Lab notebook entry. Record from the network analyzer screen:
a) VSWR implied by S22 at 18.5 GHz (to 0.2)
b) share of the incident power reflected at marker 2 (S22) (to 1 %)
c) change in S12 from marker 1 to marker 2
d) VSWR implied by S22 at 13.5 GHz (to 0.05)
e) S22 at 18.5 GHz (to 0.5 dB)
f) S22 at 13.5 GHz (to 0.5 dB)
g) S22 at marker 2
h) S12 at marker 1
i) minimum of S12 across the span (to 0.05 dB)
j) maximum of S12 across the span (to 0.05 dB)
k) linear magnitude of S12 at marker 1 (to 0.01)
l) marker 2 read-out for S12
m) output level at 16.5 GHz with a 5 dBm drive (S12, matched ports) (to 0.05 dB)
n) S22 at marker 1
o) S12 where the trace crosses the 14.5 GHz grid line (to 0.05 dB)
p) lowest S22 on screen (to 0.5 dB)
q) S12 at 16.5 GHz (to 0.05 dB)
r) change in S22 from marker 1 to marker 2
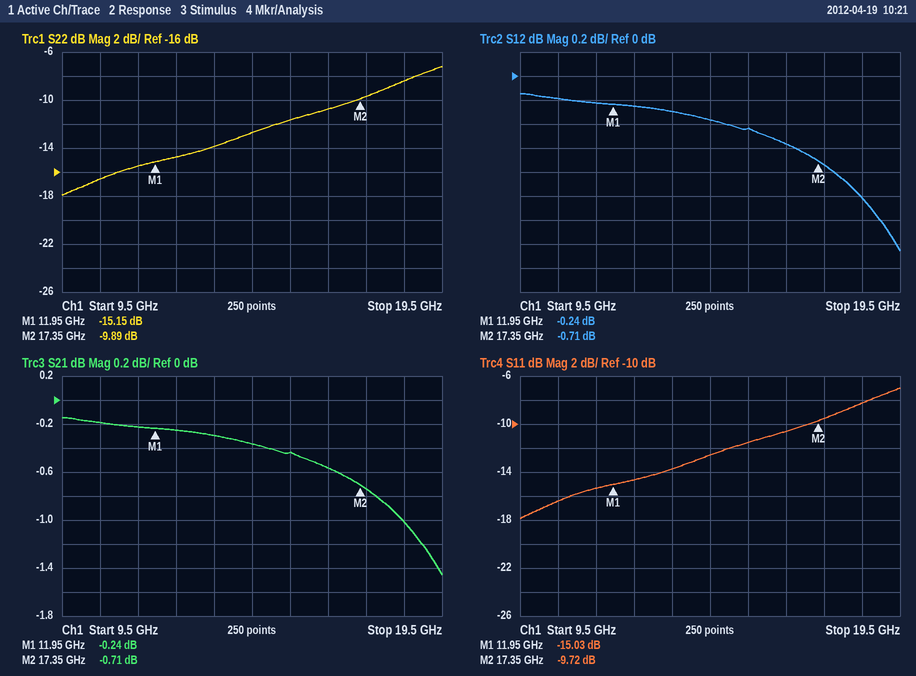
2.2
10 %
-0.47 dB
1.50
-8.5 dB
-14.0 dB
-9.89 dB
-0.24 dB
-1.45 dB
-0.15 dB
0.97
-0.71 dB
4.45 dBm
-15.15 dB
-0.35 dB
-18.0 dB
-0.55 dB
5.26 dB
